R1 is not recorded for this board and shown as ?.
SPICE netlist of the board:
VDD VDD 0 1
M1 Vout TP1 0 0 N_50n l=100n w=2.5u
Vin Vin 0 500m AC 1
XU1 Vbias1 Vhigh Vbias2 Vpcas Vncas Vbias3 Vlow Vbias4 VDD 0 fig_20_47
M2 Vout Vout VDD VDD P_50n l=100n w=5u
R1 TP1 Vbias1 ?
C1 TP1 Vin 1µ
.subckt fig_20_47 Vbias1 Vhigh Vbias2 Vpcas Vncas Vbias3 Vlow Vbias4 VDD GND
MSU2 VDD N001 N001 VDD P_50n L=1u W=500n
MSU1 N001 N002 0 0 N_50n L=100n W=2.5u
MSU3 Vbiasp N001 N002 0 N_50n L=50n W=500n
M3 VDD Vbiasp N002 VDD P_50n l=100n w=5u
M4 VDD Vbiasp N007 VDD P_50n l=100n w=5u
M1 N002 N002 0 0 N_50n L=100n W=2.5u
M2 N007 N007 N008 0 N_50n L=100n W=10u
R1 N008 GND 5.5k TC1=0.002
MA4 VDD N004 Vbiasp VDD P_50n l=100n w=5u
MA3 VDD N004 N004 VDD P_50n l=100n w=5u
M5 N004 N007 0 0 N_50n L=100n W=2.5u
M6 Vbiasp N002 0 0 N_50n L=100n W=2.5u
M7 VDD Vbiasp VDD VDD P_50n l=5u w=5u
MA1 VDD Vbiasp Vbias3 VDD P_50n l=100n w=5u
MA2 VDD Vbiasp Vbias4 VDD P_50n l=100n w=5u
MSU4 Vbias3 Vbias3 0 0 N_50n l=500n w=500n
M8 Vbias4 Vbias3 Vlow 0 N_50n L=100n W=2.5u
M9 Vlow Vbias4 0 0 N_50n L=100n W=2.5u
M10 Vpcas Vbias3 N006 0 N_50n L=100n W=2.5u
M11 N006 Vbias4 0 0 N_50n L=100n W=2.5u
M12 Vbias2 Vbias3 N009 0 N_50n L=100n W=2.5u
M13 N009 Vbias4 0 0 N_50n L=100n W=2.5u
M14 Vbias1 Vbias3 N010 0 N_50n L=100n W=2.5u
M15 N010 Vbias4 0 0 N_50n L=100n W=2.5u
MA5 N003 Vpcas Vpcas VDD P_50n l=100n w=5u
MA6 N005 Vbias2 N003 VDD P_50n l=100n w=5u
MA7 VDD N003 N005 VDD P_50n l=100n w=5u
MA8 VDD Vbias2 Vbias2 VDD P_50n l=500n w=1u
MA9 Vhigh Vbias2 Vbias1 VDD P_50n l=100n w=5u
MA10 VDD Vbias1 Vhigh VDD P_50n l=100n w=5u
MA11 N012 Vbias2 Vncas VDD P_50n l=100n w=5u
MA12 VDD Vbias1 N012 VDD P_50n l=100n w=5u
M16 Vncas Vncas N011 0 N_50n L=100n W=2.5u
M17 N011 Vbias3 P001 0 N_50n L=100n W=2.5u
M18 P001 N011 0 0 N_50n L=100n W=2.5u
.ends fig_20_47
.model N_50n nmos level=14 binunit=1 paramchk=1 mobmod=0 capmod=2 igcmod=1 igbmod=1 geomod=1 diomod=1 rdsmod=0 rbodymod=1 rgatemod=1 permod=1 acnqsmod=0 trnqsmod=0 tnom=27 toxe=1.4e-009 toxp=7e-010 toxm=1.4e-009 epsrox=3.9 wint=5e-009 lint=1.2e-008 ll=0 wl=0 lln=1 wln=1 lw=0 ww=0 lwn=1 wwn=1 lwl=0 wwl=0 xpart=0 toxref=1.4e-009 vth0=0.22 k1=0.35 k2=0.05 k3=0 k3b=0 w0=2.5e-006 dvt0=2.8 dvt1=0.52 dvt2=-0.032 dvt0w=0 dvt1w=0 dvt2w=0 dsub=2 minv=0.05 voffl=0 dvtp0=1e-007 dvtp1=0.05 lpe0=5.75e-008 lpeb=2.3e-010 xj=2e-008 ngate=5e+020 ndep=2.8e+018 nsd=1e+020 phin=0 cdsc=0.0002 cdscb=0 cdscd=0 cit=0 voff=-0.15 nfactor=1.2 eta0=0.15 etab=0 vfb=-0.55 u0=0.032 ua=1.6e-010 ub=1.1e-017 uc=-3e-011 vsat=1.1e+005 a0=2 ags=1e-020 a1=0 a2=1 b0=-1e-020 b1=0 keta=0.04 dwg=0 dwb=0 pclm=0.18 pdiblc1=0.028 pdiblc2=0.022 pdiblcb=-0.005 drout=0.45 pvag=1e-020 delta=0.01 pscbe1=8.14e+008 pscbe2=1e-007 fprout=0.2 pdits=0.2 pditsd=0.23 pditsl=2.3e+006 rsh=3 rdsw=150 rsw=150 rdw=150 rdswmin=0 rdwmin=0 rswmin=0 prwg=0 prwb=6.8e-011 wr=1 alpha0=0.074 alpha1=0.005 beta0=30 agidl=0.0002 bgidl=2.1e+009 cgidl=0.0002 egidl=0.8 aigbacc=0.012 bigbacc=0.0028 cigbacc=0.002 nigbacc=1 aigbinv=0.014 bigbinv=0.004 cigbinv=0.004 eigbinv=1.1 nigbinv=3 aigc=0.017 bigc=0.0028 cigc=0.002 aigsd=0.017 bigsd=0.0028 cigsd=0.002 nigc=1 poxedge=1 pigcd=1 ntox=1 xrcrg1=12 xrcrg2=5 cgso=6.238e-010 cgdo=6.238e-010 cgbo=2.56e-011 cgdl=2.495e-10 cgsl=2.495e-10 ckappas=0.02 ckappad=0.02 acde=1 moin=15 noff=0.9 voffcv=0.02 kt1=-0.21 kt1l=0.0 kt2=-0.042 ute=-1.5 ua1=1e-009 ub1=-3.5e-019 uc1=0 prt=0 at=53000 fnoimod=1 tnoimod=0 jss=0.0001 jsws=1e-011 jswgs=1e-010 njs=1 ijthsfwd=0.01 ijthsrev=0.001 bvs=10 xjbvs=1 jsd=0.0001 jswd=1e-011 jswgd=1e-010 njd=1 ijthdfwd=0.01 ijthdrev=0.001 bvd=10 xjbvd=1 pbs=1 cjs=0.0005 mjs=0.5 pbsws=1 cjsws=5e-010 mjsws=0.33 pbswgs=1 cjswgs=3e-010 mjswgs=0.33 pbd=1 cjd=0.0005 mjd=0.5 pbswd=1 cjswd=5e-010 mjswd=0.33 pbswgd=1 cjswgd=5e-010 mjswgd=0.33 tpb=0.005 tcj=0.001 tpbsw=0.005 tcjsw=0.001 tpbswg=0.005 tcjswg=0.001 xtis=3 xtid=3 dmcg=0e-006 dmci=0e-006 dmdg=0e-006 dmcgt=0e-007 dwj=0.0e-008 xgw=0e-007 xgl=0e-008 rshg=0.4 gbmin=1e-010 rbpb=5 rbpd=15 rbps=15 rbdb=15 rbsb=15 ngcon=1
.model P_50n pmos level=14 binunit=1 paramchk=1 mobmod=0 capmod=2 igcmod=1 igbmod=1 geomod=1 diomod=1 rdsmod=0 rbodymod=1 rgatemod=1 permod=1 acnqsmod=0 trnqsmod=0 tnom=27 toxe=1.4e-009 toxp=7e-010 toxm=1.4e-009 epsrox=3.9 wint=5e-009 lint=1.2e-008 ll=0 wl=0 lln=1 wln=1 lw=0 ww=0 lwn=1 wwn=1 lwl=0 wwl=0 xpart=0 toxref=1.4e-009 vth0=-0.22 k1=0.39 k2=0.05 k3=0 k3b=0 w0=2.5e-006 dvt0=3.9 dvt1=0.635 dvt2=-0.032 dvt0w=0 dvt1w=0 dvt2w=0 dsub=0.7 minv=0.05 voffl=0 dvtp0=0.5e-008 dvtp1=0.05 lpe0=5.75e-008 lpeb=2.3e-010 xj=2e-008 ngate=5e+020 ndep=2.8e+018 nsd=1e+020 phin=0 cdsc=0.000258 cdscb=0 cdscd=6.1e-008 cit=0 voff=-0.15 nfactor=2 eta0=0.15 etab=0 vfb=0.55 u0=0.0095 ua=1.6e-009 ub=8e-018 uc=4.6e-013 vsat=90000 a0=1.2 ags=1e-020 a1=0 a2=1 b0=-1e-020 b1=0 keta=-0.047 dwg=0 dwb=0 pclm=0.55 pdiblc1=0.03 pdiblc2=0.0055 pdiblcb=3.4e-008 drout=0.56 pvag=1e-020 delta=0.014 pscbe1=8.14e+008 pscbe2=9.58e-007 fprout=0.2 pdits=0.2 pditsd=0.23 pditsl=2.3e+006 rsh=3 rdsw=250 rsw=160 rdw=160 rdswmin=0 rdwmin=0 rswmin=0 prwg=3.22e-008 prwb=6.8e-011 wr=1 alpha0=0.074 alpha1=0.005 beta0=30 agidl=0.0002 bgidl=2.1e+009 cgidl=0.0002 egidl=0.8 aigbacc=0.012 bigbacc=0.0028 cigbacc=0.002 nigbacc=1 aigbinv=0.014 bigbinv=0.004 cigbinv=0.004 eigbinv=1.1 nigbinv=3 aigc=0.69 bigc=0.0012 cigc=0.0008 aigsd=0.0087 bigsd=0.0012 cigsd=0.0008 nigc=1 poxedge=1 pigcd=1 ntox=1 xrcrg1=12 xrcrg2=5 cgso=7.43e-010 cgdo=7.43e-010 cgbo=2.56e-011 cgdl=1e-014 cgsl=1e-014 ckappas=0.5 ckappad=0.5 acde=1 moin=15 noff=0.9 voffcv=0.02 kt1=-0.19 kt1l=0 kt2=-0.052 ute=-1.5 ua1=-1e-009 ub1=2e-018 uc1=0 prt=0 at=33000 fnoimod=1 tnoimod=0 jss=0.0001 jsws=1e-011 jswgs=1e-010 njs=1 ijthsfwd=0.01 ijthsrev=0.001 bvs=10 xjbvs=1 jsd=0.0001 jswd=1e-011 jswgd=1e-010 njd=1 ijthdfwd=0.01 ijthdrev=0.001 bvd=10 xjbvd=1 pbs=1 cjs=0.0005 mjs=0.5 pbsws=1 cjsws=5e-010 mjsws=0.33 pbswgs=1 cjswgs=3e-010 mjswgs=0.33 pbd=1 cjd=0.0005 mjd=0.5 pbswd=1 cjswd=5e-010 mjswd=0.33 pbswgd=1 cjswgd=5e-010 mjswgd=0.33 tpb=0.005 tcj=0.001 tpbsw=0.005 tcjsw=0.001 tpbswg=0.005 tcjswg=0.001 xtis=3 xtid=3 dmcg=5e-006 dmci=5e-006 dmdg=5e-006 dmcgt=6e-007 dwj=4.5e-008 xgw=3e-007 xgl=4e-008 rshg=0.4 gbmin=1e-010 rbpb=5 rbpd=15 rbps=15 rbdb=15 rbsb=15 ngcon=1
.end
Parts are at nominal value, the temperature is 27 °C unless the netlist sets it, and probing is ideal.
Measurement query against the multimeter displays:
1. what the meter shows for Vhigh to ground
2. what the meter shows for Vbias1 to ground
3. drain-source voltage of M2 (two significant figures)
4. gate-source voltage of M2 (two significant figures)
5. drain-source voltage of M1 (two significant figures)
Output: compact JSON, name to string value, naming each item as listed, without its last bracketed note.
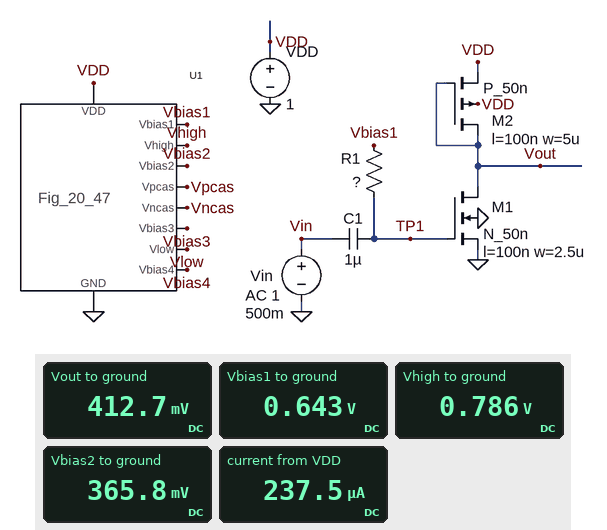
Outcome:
{"what the meter shows for Vhigh to ground": "0.786 V", "what the meter shows for Vbias1 to ground": "0.643 V", "drain-source voltage of M2": "-590 mV", "gate-source voltage of M2": "-590 mV", "drain-source voltage of M1": "410 mV"}
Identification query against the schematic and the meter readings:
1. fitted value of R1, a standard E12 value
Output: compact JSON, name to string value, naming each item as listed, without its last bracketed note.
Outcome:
{"fitted value of R1, a standard E12 value": "68 MΩ"}
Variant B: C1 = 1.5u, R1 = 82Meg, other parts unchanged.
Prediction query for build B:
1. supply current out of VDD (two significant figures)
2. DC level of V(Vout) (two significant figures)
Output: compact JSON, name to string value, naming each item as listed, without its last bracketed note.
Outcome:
{"supply current out of VDD": "230 µA", "DC level of V(Vout)": "420 mV"}
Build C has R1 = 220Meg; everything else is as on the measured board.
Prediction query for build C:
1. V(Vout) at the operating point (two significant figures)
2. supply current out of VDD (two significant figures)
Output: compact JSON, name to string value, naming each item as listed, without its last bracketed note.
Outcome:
{"V(Vout) at the operating point": "480 mV", "supply current out of VDD": "190 µA"}
